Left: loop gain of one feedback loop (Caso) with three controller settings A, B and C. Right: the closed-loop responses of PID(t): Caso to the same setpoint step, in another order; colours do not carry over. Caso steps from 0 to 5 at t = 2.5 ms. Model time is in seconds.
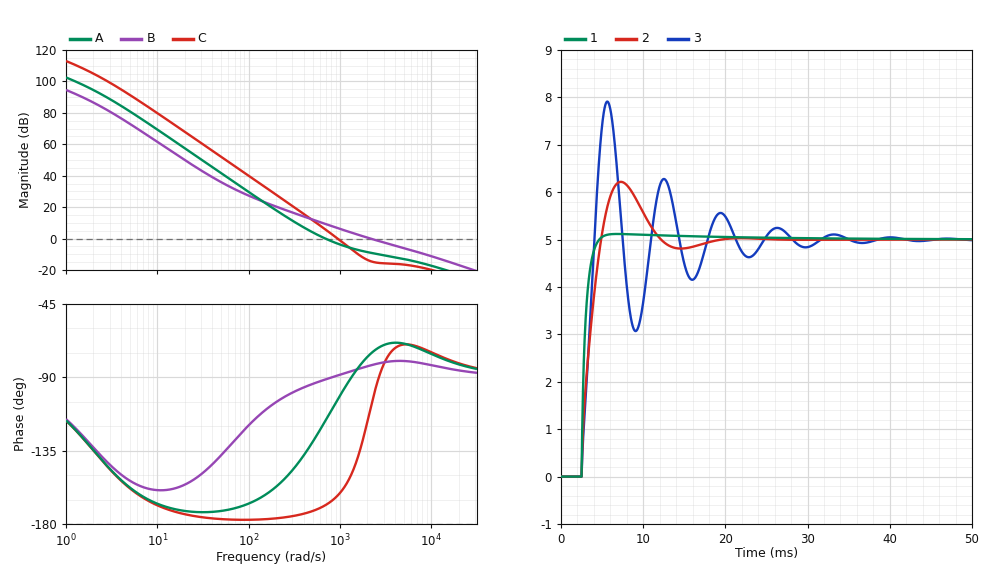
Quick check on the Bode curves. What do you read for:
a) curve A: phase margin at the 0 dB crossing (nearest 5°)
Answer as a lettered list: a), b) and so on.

a) 65°
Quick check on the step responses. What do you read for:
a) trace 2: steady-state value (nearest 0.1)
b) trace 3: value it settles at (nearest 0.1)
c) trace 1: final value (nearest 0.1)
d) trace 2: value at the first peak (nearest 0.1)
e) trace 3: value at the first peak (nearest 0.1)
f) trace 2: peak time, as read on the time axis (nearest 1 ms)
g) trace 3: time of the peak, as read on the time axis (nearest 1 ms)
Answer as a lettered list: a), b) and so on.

a) 5.0
b) 5.0
c) 5.0
d) 6.2
e) 7.9
f) 7 ms
g) 6 ms
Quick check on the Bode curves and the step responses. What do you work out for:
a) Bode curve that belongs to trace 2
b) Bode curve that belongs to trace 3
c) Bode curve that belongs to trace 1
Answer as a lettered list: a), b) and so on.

a) A
b) C
c) B
